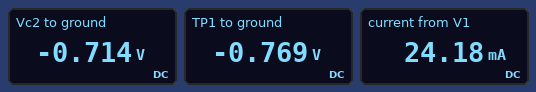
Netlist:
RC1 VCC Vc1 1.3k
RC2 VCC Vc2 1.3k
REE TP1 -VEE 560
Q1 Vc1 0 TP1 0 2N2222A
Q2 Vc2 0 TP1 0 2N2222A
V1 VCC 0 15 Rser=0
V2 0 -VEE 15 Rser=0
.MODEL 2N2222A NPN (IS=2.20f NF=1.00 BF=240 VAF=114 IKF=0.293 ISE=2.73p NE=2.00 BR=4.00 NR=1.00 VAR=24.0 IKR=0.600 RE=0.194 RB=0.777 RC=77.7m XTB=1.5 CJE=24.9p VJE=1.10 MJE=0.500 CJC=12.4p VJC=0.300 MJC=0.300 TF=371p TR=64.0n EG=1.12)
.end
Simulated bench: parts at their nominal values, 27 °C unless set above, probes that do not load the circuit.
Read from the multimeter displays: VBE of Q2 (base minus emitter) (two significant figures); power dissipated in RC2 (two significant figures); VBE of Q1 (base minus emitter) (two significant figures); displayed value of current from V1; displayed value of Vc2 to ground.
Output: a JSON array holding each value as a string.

["770 mV", "190 mW", "770 mV", "24.18 mA", "-0.714 V"]
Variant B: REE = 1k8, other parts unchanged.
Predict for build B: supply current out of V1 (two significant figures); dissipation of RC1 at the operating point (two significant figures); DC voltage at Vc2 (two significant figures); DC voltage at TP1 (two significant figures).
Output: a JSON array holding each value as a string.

["7.9 mA", "20 mW", "9.9 V", "-730 mV"]
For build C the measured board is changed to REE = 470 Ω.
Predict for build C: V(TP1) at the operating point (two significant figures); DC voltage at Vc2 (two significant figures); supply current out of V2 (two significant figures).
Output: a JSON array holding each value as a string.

["-790 mV", "-760 mV", "30 mA"]
